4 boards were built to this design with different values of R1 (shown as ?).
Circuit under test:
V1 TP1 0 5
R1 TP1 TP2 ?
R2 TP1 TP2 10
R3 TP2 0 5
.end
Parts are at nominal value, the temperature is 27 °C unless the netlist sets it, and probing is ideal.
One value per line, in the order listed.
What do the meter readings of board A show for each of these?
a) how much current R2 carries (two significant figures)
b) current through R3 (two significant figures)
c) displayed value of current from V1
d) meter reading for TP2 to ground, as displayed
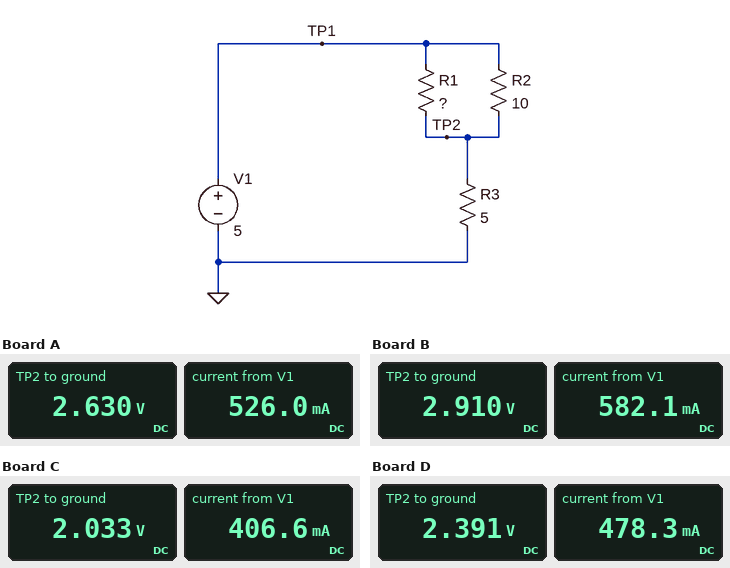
240 mA
530 mA
526.0 mA
2.630 V
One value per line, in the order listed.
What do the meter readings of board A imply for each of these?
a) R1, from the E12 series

8.2 Ω
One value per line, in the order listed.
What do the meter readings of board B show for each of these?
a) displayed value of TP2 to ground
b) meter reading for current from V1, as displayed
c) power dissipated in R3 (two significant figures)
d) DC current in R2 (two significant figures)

2.910 V
582.1 mA
1.7 W
210 mA
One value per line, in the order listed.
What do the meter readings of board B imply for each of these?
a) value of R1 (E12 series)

5.6 Ω
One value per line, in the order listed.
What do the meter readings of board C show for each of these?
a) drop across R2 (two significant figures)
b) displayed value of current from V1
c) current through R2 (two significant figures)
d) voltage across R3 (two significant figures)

3.0 V
406.6 mA
300 mA
2.0 V
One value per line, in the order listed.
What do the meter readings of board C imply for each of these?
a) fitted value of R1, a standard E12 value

27 Ω
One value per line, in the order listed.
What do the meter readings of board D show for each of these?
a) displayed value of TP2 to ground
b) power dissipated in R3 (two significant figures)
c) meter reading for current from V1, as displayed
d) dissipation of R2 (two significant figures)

2.391 V
1.1 W
478.3 mA
680 mW
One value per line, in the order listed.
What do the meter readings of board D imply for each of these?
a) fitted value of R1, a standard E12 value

12 Ω
